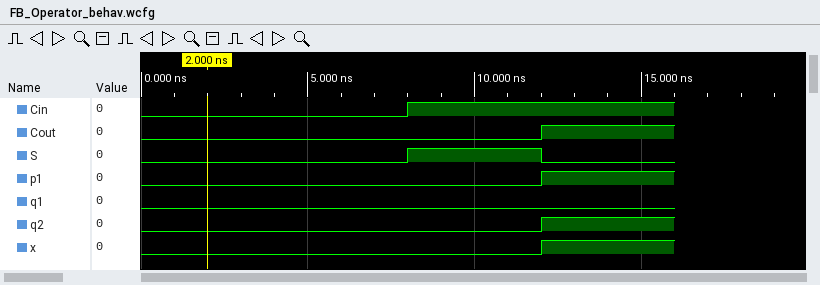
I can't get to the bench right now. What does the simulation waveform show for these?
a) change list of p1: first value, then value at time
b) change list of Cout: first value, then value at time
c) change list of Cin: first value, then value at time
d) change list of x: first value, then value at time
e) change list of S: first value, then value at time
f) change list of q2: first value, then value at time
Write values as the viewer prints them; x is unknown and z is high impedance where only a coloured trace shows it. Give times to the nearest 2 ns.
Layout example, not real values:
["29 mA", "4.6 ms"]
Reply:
["0, 1 at 12 ns", "0, 1 at 12 ns", "0, 1 at 8 ns", "0, 1 at 12 ns", "0, 1 at 8 ns, 0 at 12 ns", "0, 1 at 12 ns"]
